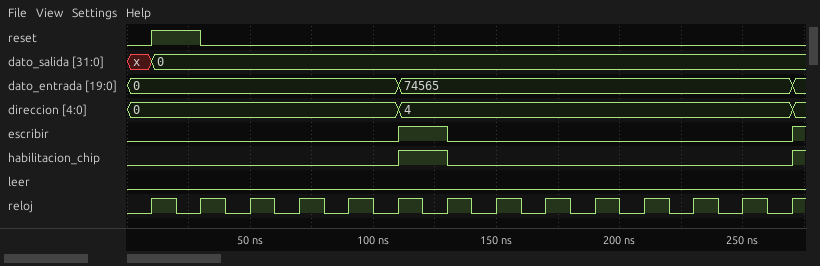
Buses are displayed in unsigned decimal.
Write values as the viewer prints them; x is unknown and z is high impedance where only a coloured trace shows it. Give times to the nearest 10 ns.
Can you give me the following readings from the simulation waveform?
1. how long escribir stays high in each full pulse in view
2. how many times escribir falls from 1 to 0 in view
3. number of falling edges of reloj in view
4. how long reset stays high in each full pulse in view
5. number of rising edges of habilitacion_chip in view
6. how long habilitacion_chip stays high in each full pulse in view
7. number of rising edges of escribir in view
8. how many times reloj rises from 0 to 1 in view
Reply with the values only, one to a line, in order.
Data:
20 ns
1
13
20 ns
2
20 ns
2
14
